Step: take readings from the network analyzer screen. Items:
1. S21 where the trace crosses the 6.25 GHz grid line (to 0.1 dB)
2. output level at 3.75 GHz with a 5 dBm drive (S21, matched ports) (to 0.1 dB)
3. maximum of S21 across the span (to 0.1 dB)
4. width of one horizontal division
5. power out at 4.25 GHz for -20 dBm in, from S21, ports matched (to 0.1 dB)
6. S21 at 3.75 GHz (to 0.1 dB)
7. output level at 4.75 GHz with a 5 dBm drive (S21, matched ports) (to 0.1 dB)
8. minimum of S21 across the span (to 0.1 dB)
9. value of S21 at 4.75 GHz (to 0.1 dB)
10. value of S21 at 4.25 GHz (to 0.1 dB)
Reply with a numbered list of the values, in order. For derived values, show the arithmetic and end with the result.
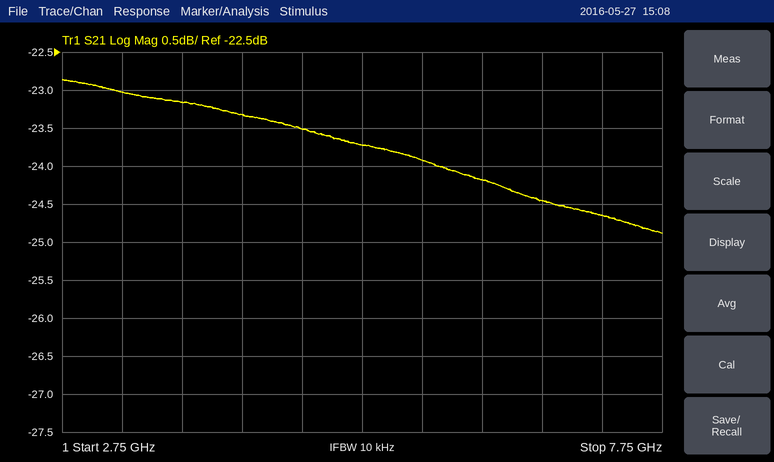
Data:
1. -24.2 dB
2. 5 dBm + (-23.2 dB) = -18.2 dBm
3. -22.9 dB
4. 500 MHz
5. -20 dBm + (-23.3 dB) = -43.3 dBm
6. -23.2 dB
7. 5 dBm + (-23.5 dB) = -18.5 dBm
8. -24.9 dB
9. -23.5 dB
10. -23.3 dB
